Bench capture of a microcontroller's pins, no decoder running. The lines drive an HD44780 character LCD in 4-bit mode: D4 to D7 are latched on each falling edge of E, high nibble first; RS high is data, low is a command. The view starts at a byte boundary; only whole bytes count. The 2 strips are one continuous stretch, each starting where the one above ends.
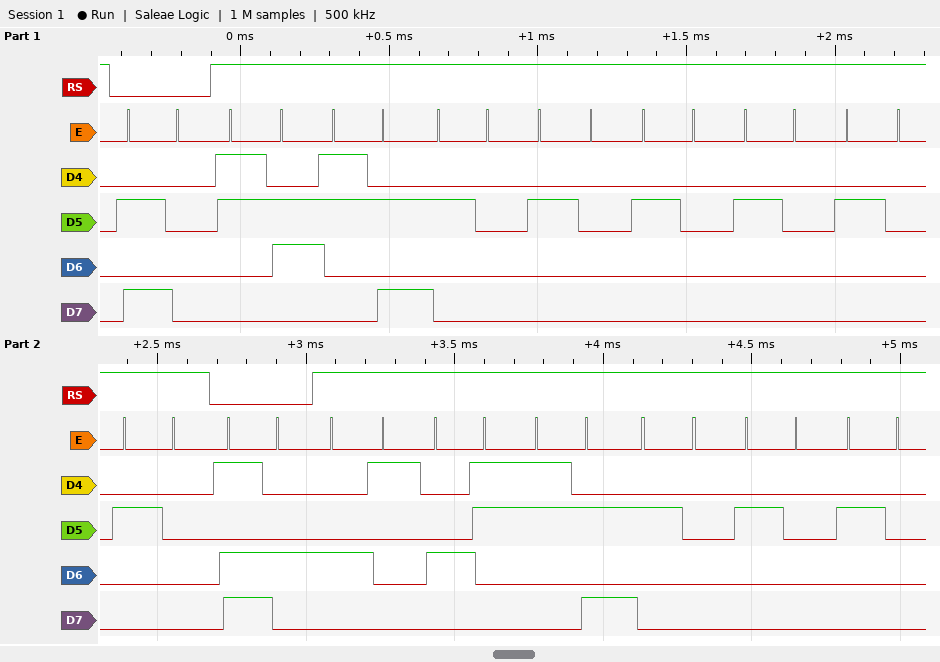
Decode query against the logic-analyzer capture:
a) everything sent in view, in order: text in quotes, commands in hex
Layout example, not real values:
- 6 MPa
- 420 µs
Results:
- 0xA0 "6:      " 0xD4 "AC:   "
